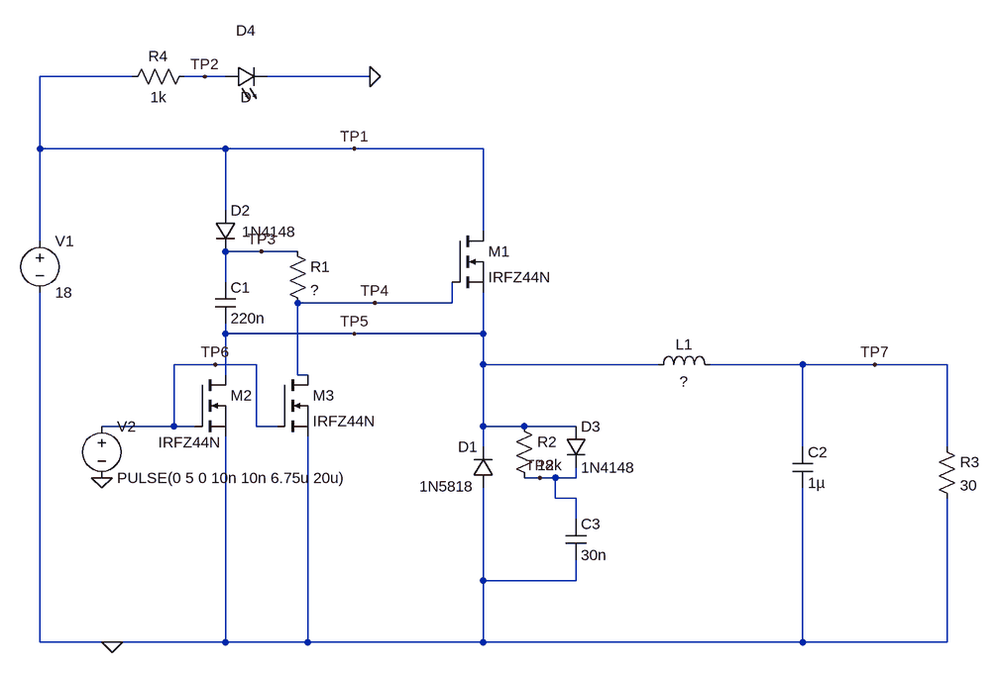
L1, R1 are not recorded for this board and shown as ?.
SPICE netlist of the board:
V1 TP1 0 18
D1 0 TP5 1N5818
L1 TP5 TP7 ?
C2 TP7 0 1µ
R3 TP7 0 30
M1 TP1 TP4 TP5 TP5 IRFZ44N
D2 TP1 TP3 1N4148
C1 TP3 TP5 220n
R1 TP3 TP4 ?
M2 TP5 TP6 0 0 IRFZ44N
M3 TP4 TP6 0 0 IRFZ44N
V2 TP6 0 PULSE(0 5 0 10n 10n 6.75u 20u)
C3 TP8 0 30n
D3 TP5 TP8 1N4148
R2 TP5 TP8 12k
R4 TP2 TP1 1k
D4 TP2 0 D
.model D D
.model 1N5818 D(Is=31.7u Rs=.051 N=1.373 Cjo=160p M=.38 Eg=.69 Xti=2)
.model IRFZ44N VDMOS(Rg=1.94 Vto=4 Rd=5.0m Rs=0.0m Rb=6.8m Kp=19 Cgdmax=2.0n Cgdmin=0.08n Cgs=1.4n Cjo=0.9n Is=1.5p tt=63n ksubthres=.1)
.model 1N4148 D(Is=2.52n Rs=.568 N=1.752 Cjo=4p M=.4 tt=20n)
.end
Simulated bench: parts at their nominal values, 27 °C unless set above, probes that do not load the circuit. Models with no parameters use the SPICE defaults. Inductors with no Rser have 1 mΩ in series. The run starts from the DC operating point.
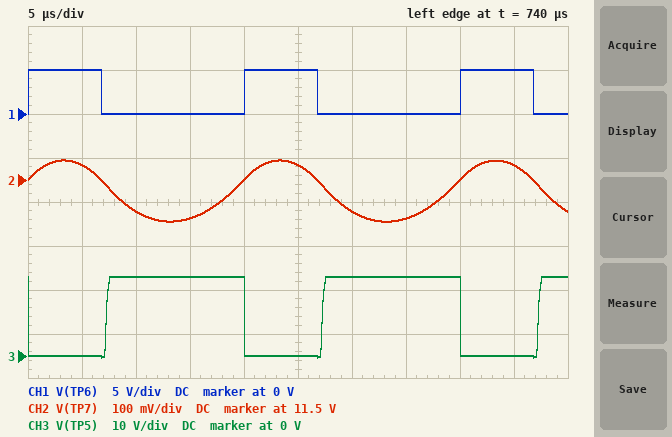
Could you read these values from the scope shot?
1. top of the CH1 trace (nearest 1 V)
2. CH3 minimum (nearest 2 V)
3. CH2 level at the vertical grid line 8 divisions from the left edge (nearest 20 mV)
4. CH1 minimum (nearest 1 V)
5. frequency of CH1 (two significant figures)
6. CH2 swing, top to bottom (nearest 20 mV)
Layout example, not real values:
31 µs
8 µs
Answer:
5 V
0 V
11.50 V
0 V
50 kHz
140 mV
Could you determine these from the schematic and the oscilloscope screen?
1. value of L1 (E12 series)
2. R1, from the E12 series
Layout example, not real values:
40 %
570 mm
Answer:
1.5 mH
330 Ω
